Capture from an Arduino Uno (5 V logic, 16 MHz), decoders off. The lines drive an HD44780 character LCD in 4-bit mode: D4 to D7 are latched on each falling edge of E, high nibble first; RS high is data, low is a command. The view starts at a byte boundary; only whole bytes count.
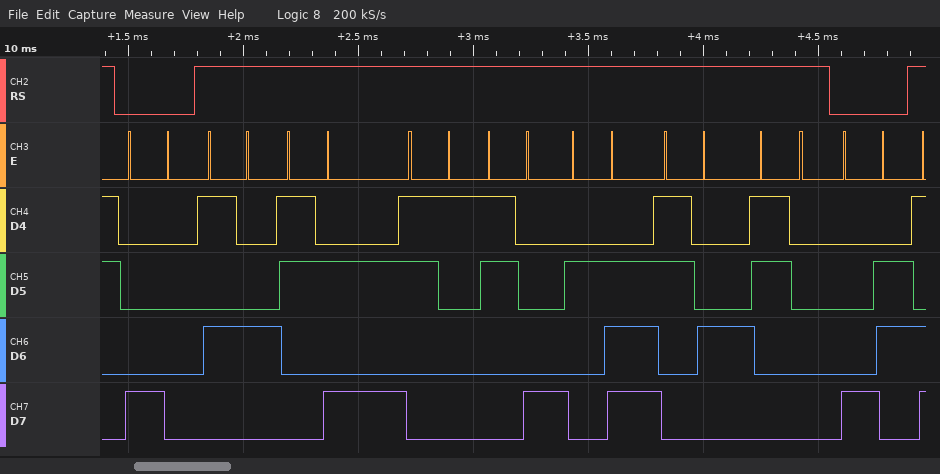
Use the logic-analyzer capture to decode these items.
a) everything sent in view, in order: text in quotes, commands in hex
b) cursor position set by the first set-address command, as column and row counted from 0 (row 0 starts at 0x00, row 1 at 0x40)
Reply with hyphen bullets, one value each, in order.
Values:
- 0x80 "T:18.40" 0x86
- column 0, row 0
